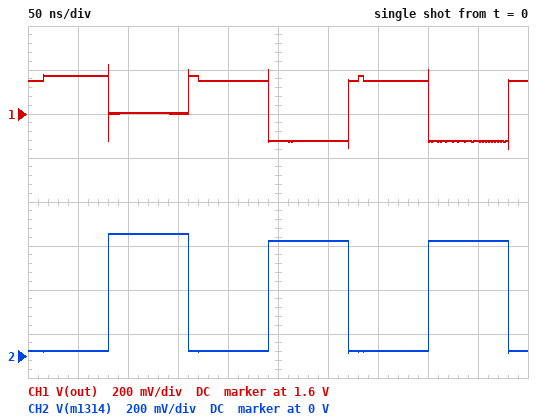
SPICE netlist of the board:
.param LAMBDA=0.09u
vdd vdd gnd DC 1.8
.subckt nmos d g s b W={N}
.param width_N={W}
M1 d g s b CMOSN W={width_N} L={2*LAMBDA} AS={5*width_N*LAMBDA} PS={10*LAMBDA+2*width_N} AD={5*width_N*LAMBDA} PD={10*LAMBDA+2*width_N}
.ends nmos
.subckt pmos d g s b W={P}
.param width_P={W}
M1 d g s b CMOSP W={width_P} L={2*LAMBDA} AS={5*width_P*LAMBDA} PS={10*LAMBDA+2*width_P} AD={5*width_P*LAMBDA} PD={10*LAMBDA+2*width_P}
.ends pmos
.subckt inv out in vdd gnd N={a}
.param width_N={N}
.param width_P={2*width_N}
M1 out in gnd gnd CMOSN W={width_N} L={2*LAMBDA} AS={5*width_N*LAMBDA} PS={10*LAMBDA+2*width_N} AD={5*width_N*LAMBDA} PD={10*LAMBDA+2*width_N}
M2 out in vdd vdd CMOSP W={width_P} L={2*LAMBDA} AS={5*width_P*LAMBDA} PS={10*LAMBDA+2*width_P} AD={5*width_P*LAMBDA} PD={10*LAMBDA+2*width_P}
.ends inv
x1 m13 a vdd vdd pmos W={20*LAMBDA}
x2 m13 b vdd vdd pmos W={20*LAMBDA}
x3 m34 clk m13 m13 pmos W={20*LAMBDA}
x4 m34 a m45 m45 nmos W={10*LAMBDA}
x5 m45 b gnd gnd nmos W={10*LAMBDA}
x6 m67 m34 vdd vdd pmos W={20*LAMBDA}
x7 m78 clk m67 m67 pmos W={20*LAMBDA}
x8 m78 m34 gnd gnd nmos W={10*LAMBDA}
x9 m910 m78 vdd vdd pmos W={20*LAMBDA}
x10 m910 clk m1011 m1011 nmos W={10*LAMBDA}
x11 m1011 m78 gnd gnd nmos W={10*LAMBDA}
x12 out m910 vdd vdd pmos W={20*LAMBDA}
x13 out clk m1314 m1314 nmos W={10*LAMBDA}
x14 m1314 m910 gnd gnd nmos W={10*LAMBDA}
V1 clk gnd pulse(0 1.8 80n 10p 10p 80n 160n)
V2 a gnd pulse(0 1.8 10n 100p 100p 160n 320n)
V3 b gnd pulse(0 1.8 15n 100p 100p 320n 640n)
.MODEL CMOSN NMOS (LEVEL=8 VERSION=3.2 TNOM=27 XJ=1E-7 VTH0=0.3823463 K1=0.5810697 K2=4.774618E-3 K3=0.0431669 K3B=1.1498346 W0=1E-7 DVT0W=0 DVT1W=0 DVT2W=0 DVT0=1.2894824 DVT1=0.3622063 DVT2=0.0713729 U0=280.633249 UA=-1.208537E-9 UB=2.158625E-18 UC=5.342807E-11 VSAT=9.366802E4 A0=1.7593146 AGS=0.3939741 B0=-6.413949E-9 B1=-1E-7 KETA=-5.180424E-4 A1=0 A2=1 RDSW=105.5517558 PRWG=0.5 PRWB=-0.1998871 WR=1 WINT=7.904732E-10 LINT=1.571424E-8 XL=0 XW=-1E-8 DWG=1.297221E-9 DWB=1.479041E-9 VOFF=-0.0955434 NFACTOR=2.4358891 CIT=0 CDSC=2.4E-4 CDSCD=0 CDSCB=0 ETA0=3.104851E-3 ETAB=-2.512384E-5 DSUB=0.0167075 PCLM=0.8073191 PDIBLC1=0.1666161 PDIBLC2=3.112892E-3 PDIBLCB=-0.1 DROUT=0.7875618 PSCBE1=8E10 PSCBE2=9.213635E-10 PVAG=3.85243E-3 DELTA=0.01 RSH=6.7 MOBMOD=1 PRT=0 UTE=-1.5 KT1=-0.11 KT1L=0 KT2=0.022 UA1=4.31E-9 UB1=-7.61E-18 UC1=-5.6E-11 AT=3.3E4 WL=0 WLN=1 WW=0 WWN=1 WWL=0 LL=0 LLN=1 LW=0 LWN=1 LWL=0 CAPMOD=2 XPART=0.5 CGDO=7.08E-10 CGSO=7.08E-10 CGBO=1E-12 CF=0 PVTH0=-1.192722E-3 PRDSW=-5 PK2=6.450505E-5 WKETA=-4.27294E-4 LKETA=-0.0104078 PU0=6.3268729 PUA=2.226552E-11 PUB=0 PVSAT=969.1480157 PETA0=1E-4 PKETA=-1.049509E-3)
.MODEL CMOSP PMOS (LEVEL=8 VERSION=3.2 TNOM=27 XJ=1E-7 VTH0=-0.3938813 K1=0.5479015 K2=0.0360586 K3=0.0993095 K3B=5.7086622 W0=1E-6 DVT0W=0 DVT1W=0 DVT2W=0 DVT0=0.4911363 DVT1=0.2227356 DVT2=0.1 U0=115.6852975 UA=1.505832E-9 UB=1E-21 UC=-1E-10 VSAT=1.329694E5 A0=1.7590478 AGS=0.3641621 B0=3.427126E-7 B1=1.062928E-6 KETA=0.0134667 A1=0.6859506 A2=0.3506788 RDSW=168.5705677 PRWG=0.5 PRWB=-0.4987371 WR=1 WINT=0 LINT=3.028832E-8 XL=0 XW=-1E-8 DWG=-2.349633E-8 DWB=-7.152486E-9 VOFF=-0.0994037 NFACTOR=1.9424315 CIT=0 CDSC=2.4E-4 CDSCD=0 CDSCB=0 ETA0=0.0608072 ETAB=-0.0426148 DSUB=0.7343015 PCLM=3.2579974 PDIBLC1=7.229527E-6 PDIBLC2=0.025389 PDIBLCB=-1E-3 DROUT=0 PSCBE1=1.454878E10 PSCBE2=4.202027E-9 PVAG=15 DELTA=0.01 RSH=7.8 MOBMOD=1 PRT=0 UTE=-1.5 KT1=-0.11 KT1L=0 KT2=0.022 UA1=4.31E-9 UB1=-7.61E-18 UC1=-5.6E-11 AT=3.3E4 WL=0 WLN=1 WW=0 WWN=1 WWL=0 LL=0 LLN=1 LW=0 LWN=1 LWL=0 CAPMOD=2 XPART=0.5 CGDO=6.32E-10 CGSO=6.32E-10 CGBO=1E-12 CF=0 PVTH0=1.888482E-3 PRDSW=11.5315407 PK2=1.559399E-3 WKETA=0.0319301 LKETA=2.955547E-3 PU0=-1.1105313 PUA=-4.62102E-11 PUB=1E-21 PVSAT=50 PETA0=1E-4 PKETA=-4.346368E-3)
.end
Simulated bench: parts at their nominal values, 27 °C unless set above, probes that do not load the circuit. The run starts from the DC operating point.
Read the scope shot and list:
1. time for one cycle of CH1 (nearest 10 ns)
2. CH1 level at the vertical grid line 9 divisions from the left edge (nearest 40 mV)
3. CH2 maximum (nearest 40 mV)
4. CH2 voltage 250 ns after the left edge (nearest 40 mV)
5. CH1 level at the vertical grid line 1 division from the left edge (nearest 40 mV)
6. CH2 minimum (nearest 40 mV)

160 ns
1.48 V
560 mV
520 mV
1.76 V
0 V
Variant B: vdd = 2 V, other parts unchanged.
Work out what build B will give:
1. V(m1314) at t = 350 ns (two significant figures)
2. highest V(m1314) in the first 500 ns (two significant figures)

34 mV
540 mV
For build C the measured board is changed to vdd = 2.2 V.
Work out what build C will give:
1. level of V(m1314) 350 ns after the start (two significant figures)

48 mV
